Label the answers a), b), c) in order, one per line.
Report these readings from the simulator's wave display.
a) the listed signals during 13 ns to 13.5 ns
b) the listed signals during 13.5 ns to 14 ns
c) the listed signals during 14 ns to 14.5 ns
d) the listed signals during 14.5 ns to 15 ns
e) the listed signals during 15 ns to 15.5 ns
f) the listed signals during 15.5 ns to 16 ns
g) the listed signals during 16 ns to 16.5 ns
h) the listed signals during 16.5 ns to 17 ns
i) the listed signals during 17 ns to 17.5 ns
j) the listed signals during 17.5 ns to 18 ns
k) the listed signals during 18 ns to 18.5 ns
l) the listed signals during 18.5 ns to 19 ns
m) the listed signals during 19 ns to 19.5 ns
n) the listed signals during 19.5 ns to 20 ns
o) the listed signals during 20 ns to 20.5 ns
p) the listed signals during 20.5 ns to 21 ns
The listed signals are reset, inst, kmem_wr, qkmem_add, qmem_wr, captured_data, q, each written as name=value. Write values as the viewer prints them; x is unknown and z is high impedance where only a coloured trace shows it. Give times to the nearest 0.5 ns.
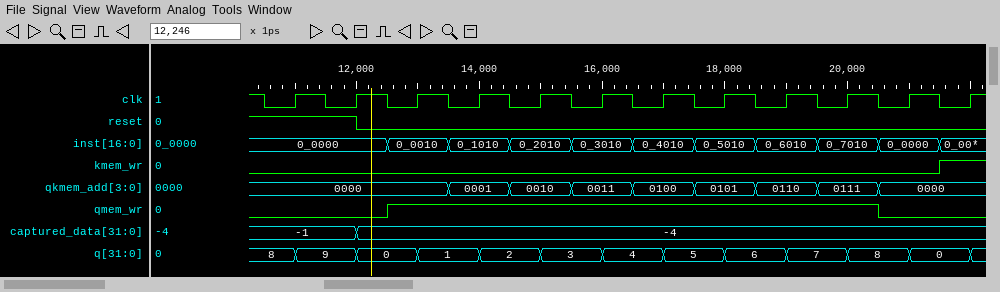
a) reset=0, inst=0_0010, kmem_wr=0, qkmem_add=0000, qmem_wr=1, captured_data=-4, q=1
b) reset=0, inst=0_1010, kmem_wr=0, qkmem_add=0001, qmem_wr=1, captured_data=-4, q=1
c) reset=0, inst=0_1010, kmem_wr=0, qkmem_add=0001, qmem_wr=1, captured_data=-4, q=2
d) reset=0, inst=0_2010, kmem_wr=0, qkmem_add=0010, qmem_wr=1, captured_data=-4, q=2
e) reset=0, inst=0_2010, kmem_wr=0, qkmem_add=0010, qmem_wr=1, captured_data=-4, q=3
f) reset=0, inst=0_3010, kmem_wr=0, qkmem_add=0011, qmem_wr=1, captured_data=-4, q=3
g) reset=0, inst=0_3010, kmem_wr=0, qkmem_add=0011, qmem_wr=1, captured_data=-4, q=4
h) reset=0, inst=0_4010, kmem_wr=0, qkmem_add=0100, qmem_wr=1, captured_data=-4, q=4
i) reset=0, inst=0_4010, kmem_wr=0, qkmem_add=0100, qmem_wr=1, captured_data=-4, q=5
j) reset=0, inst=0_5010, kmem_wr=0, qkmem_add=0101, qmem_wr=1, captured_data=-4, q=5
k) reset=0, inst=0_5010, kmem_wr=0, qkmem_add=0101, qmem_wr=1, captured_data=-4, q=6
l) reset=0, inst=0_6010, kmem_wr=0, qkmem_add=0110, qmem_wr=1, captured_data=-4, q=6
m) reset=0, inst=0_6010, kmem_wr=0, qkmem_add=0110, qmem_wr=1, captured_data=-4, q=7
n) reset=0, inst=0_7010, kmem_wr=0, qkmem_add=0111, qmem_wr=1, captured_data=-4, q=7
o) reset=0, inst=0_7010, kmem_wr=0, qkmem_add=0111, qmem_wr=1, captured_data=-4, q=8
p) reset=0, inst=0_0000, kmem_wr=0, qkmem_add=0000, qmem_wr=0, captured_data=-4, q=8
